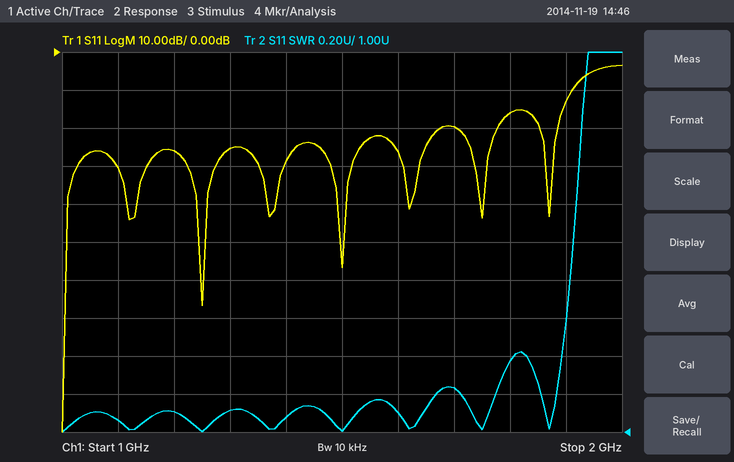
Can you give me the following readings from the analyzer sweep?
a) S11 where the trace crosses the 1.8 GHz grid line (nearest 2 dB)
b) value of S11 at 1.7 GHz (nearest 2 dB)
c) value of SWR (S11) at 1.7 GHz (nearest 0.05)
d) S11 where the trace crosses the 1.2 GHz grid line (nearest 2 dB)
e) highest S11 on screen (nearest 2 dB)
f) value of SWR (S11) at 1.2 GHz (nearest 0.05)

-16 dB
-20 dB
1.25
-26 dB
-4 dB
1.10
